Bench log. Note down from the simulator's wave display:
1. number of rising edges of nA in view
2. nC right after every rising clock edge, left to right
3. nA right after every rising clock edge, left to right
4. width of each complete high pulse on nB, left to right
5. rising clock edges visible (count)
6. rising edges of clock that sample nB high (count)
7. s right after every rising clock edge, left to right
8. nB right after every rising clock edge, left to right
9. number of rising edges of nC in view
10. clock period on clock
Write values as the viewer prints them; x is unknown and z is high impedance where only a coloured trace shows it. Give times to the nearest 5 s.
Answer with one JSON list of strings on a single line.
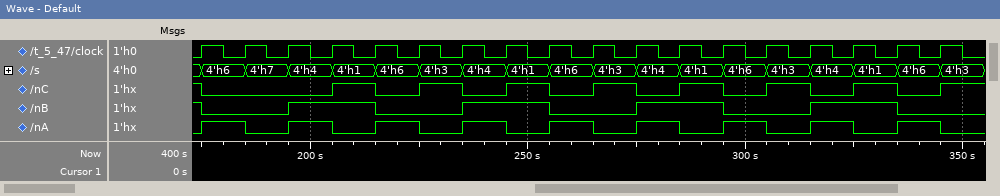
["9", "0 0 0 1 0 1 0 1 0 1 0 1 0 1 0 1 0 1", "1 0 1 0 1 0 1 0 1 0 1 0 1 0 1 0 1 0", "20 s, 20 s, 20 s, 20 s", "18", "9", "4'h6, 4'h7, 4'h4, 4'h1, 4'h6, 4'h3, 4'h4, 4'h1, 4'h6, 4'h3, 4'h4, 4'h1, 4'h6, 4'h3, 4'h4, 4'h1, 4'h6, 4'h3", "0 0 1 1 0 0 1 1 0 0 1 1 0 0 1 1 0 0", "8", "10 s"]
